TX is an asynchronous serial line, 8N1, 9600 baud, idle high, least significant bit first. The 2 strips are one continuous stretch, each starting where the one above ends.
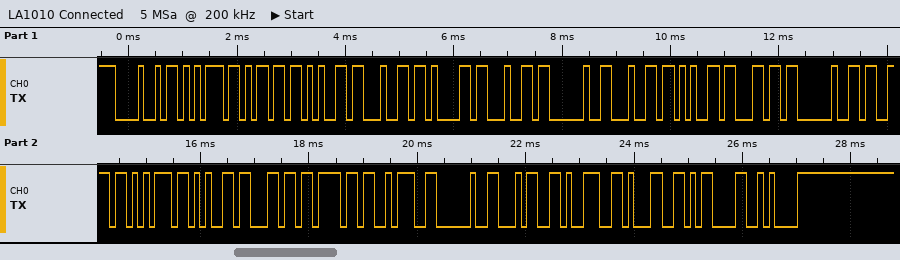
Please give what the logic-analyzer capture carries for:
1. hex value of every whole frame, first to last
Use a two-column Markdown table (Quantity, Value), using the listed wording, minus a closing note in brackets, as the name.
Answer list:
| Quantity | Value |
|---|---|
| hex value of every whole frame, first to last | 48 75 6D 65 64 61 64 20 64 65 6C 20 73 75 65 6C 6F 3A 20 34 39 31 0D 0A |
